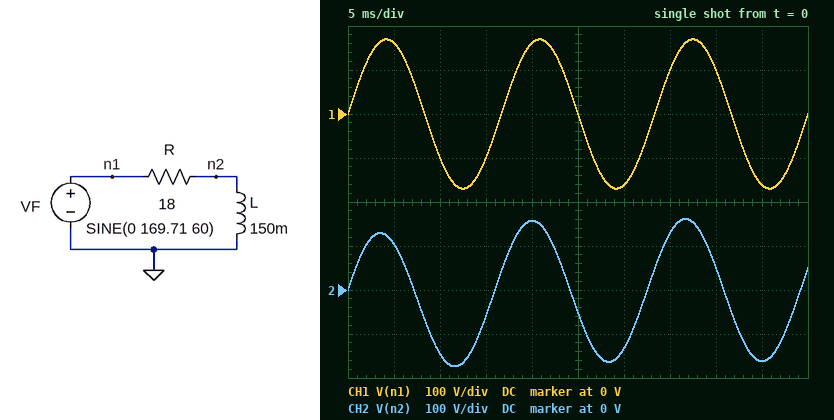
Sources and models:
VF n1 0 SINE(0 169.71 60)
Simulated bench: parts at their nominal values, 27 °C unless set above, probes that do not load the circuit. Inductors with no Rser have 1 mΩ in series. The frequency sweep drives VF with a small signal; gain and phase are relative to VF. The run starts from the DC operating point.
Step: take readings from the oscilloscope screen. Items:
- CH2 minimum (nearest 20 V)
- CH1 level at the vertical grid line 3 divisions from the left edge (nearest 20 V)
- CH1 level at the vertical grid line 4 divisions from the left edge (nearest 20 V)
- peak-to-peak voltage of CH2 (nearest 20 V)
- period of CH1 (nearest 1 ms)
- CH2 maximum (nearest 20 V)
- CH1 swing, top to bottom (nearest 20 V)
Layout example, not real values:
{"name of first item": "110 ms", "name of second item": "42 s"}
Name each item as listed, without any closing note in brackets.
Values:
{"CH2 minimum": "-180 V", "CH1 level at the vertical grid line 3 divisions from the left edge": "-100 V", "CH1 level at the vertical grid line 4 divisions from the left edge": "160 V", "peak-to-peak voltage of CH2": "340 V", "period of CH1": "17 ms", "CH2 maximum": "160 V", "CH1 swing, top to bottom": "340 V"}
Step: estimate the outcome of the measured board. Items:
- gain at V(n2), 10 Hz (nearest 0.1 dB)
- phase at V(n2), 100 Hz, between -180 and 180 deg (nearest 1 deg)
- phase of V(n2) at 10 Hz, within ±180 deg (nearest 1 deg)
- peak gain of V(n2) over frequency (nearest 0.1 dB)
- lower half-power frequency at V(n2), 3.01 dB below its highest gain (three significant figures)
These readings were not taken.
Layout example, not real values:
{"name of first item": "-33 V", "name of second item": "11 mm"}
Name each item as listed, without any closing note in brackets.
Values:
{"gain at V(n2), 10 Hz": "-6.7 dB", "phase at V(n2), 100 Hz, between -180 and 180 deg": "11 deg", "phase of V(n2) at 10 Hz, within ±180 deg": "62 deg", "peak gain of V(n2) over frequency": "0 dB", "lower half-power frequency at V(n2), 3.01 dB below its highest gain": "19.1 Hz"}
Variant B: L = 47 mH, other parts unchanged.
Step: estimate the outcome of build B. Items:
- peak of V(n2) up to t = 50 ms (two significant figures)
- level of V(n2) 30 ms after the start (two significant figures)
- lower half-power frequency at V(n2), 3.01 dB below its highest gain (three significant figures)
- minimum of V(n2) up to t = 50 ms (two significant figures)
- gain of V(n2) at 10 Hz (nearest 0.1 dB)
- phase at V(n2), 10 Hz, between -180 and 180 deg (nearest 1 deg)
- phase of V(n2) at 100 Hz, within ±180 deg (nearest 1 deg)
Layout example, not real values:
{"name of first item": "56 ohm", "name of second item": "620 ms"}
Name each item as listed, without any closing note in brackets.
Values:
{"peak of V(n2) up to t = 50 ms": "120 V", "level of V(n2) 30 ms after the start": "-53 V", "lower half-power frequency at V(n2), 3.01 dB below its highest gain": "61.0 Hz", "minimum of V(n2) up to t = 50 ms": "-120 V", "gain of V(n2) at 10 Hz": "-15.8 dB", "phase at V(n2), 10 Hz, between -180 and 180 deg": "81 deg", "phase of V(n2) at 100 Hz, within ±180 deg": "31 deg"}
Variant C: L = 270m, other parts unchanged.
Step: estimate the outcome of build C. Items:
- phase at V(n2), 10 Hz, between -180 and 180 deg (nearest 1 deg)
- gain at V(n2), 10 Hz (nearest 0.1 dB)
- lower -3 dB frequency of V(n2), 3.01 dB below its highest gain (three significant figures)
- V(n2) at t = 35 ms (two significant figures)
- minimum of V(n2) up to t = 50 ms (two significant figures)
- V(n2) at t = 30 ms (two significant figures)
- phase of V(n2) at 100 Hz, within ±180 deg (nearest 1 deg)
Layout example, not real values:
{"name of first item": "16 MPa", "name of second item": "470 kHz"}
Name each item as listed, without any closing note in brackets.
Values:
{"phase at V(n2), 10 Hz, between -180 and 180 deg": "47 deg", "gain at V(n2), 10 Hz": "-3.3 dB", "lower -3 dB frequency of V(n2), 3.01 dB below its highest gain": "10.6 Hz", "V(n2) at t = 35 ms": "120 V", "minimum of V(n2) up to t = 50 ms": "-180 V", "V(n2) at t = 30 ms": "-150 V", "phase of V(n2) at 100 Hz, within ±180 deg": "6 deg"}
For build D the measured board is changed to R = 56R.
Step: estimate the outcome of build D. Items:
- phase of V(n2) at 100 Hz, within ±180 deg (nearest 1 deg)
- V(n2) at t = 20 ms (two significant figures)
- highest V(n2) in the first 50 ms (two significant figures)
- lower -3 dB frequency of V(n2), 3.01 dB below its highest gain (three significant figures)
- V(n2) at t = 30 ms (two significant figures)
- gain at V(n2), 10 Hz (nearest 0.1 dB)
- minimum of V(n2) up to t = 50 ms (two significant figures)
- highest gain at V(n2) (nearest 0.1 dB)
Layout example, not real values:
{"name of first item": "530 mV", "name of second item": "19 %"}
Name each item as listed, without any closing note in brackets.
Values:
{"phase of V(n2) at 100 Hz, within ±180 deg": "31 deg", "V(n2) at t = 20 ms": "110 V", "highest V(n2) in the first 50 ms": "120 V", "lower -3 dB frequency of V(n2), 3.01 dB below its highest gain": "59.4 Hz", "V(n2) at t = 30 ms": "-55 V", "gain at V(n2), 10 Hz": "-15.6 dB", "minimum of V(n2) up to t = 50 ms": "-120 V", "highest gain at V(n2)": "0 dB"}
